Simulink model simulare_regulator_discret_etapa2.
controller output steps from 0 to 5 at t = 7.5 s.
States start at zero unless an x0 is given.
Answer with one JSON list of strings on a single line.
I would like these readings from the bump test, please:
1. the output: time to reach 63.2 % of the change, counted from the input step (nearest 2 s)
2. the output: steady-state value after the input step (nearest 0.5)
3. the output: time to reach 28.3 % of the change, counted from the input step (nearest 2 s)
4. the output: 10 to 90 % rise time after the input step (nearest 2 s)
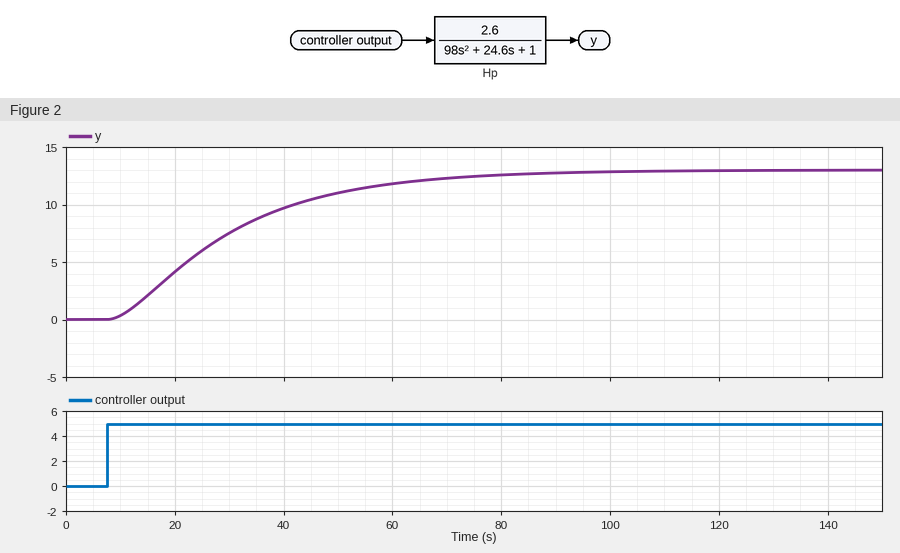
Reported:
["26 s", "13.0", "12 s", "46 s"]
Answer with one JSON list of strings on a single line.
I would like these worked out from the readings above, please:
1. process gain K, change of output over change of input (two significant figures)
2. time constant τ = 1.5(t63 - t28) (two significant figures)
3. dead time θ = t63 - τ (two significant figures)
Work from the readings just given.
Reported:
["2.6", "21 s", "5.0 s"]
